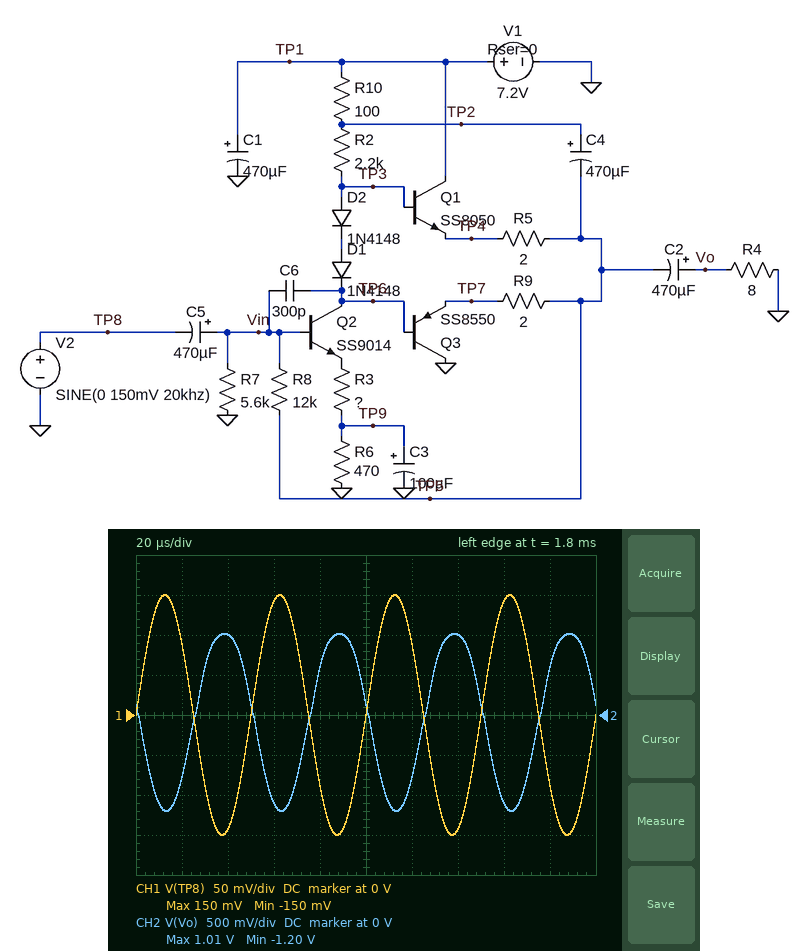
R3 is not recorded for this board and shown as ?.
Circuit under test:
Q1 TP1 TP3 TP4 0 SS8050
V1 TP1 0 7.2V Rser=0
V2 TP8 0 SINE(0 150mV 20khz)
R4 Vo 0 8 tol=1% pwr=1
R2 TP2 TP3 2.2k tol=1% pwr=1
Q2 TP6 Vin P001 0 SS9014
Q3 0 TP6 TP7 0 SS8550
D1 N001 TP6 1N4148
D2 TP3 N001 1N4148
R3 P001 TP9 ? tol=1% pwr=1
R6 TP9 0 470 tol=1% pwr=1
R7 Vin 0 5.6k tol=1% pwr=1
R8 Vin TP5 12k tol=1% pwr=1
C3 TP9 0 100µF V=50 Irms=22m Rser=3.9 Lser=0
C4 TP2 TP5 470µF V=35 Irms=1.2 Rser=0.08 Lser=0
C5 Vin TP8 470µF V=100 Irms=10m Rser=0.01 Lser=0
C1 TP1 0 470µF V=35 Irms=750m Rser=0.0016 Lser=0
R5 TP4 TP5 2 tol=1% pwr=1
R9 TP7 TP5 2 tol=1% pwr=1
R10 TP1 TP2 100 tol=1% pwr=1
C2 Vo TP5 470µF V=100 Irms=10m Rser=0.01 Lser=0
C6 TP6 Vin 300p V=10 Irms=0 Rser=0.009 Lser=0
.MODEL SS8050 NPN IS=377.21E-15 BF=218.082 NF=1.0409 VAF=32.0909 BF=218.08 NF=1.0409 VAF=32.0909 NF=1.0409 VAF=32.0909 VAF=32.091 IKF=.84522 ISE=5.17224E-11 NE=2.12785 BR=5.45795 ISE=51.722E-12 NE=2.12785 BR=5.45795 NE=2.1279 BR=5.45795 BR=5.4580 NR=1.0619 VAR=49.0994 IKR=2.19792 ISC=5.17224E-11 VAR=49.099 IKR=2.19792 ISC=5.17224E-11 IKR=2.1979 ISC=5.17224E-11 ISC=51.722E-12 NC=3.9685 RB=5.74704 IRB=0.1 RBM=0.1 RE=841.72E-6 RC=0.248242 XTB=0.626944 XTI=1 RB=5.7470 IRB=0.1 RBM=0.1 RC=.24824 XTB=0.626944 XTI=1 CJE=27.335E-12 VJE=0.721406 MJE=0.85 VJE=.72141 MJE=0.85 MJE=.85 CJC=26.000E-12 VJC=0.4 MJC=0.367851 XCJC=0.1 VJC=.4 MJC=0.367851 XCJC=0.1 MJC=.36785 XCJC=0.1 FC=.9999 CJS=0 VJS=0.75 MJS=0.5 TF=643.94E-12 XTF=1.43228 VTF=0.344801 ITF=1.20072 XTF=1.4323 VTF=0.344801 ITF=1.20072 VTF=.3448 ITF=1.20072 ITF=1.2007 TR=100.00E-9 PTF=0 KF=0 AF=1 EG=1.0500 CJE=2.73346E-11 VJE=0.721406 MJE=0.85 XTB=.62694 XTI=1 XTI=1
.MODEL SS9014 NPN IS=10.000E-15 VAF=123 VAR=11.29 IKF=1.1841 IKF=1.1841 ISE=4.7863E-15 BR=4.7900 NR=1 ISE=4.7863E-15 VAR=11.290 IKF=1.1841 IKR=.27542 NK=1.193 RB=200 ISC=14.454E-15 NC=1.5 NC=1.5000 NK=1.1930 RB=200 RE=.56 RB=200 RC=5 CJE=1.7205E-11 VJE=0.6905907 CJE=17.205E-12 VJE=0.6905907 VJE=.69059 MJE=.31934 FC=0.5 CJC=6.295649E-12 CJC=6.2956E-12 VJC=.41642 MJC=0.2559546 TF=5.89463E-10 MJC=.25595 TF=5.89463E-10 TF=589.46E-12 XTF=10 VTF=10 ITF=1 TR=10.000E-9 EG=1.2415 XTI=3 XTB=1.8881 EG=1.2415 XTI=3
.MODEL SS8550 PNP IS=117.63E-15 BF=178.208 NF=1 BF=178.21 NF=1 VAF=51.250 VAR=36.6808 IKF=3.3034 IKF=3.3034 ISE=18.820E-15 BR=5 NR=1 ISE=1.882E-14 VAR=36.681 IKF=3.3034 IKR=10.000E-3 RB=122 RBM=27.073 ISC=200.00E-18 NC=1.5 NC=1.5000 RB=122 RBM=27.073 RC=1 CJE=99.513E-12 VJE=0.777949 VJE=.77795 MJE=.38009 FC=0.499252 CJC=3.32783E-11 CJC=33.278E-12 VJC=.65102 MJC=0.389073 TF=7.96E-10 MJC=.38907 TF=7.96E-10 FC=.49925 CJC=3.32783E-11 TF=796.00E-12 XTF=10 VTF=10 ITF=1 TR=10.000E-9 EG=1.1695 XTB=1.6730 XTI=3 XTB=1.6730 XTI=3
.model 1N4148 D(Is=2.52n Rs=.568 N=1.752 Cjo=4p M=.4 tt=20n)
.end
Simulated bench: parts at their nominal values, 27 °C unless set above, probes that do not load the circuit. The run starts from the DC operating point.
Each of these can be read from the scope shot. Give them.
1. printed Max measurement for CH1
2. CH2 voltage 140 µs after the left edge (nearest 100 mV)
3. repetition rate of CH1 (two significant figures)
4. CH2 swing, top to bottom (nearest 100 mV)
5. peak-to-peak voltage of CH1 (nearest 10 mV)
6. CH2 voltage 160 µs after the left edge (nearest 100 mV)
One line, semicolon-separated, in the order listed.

150 mV; 1.0 V; 20 kHz; 2.2 V; 300 mV; -1.1 V
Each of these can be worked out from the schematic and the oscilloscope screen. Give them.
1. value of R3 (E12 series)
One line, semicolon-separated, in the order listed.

100 Ω
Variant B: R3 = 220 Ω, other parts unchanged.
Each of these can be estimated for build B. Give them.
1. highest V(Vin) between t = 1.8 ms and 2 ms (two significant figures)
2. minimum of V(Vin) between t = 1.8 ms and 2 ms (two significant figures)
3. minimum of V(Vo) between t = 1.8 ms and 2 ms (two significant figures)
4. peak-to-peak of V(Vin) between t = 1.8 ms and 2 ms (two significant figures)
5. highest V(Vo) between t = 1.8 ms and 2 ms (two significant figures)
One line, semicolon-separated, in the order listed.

1.5 V; 1.2 V; -600 mV; 300 mV; 620 mV
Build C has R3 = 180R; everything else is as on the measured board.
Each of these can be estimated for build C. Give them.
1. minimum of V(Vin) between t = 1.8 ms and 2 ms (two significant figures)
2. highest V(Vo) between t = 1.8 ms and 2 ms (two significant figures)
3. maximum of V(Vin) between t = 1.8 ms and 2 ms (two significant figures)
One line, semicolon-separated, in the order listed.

1.2 V; 720 mV; 1.5 V
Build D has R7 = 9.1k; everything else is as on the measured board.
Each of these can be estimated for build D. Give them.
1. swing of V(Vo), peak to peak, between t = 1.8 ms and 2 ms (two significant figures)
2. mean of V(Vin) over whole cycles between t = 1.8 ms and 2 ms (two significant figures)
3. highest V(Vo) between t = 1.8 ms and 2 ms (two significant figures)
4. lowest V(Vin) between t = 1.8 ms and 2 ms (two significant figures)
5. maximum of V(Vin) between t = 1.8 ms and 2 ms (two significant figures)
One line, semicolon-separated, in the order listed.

2.3 V; 1.4 V; 1.1 V; 1.3 V; 1.6 V
